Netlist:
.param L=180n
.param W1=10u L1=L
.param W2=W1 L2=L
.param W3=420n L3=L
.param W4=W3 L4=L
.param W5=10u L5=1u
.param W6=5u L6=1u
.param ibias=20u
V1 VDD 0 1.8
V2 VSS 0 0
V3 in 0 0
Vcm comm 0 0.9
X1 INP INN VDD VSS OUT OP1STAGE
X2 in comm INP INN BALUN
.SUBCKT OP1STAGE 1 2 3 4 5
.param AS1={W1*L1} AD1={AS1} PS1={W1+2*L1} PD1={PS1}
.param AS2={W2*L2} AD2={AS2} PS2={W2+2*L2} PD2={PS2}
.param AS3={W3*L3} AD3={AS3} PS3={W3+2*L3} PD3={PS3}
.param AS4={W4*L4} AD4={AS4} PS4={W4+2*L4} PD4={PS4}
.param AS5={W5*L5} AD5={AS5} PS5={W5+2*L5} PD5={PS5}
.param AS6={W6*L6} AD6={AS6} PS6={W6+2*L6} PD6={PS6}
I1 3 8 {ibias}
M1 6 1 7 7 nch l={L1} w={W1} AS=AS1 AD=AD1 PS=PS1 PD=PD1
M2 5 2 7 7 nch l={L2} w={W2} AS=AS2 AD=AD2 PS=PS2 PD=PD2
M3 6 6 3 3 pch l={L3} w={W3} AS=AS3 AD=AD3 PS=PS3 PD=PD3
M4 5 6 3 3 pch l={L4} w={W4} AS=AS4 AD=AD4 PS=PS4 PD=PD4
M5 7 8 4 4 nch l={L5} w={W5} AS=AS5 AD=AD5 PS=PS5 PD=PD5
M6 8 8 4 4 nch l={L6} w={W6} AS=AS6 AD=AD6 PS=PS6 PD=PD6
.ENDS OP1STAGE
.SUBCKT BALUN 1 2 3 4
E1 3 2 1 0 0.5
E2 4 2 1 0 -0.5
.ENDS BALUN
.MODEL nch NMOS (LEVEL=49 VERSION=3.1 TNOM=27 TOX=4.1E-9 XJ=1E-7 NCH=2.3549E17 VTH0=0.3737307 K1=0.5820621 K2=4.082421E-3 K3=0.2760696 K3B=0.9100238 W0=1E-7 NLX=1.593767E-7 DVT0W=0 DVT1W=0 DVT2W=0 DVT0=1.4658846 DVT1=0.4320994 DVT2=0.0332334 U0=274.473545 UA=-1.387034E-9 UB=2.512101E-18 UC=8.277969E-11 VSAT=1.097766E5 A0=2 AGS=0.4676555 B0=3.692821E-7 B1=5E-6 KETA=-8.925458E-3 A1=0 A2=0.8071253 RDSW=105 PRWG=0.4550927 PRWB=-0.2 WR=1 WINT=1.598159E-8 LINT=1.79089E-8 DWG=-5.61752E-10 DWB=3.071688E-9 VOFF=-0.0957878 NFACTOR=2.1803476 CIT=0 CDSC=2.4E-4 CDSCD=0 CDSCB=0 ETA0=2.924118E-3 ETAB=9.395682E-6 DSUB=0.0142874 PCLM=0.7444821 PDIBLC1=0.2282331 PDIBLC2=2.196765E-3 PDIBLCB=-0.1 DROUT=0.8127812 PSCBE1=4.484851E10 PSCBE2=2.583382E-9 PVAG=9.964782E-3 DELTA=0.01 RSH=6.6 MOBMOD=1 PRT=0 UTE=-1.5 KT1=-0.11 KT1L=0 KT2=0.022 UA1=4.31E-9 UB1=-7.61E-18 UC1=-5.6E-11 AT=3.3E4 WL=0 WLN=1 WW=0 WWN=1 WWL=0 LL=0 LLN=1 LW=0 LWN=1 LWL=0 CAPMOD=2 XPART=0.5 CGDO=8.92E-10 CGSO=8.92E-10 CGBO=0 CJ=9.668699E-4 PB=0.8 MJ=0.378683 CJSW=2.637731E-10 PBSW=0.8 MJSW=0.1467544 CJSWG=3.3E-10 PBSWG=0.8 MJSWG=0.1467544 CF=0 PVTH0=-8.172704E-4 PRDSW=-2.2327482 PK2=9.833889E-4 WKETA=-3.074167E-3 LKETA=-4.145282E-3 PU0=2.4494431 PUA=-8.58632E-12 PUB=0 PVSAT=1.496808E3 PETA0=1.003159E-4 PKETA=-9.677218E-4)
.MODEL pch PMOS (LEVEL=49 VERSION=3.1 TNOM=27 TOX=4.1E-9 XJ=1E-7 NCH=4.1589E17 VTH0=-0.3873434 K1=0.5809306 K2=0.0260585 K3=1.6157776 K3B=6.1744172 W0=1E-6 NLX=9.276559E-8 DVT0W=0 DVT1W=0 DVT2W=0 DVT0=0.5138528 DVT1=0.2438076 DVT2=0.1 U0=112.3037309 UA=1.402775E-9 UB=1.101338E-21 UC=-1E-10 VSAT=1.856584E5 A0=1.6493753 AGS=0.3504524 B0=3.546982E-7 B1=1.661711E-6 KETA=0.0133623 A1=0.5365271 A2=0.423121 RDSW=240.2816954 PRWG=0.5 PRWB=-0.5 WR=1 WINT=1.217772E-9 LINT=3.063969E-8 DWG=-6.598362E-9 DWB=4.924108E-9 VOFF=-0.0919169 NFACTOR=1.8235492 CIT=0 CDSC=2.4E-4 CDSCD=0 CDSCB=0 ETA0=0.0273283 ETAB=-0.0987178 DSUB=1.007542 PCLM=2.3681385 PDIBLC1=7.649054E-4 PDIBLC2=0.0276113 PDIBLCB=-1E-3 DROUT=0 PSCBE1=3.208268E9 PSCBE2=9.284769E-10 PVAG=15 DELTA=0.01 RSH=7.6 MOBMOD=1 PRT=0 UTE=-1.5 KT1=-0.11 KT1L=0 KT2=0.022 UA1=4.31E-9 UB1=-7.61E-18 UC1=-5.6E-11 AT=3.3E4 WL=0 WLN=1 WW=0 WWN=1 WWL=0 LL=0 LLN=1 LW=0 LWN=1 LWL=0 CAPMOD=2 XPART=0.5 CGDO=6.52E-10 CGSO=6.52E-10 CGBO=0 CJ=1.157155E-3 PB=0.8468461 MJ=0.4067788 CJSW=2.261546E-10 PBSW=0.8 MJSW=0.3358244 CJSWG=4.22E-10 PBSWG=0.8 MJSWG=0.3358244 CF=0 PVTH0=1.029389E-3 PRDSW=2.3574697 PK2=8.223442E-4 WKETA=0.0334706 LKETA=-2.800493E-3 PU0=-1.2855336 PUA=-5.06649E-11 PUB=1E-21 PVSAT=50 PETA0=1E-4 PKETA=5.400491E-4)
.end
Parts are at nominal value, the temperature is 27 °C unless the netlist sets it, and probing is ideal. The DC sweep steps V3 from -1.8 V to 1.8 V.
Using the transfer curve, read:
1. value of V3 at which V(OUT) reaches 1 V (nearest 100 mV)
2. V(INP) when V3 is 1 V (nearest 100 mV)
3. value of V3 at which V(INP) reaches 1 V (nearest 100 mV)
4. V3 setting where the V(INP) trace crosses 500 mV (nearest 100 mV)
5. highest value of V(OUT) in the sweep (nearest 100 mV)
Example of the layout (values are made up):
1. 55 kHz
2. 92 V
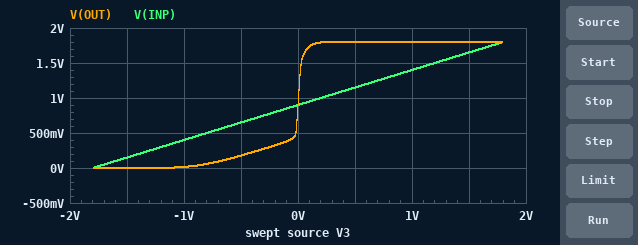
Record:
1. 0 V
2. 1.4 V
3. 200 mV
4. -800 mV
5. 1.8 V
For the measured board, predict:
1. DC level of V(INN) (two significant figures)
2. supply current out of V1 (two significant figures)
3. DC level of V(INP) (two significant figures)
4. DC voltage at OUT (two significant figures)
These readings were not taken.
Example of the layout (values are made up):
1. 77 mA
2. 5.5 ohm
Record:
1. 900 mV
2. 59 µA
3. 900 mV
4. 900 mV
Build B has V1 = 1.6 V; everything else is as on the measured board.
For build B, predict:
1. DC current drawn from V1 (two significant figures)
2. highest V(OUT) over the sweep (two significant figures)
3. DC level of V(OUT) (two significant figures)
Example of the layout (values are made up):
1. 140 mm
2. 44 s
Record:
1. 59 µA
2. 1.6 V
3. 700 mV
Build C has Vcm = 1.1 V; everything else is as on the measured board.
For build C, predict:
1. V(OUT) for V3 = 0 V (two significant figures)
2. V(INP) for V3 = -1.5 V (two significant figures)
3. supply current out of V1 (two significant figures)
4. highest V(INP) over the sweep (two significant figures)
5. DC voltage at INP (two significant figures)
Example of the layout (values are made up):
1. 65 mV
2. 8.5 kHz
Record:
1. 890 mV
2. 350 mV
3. 60 µA
4. 2.0 V
5. 1.1 V
